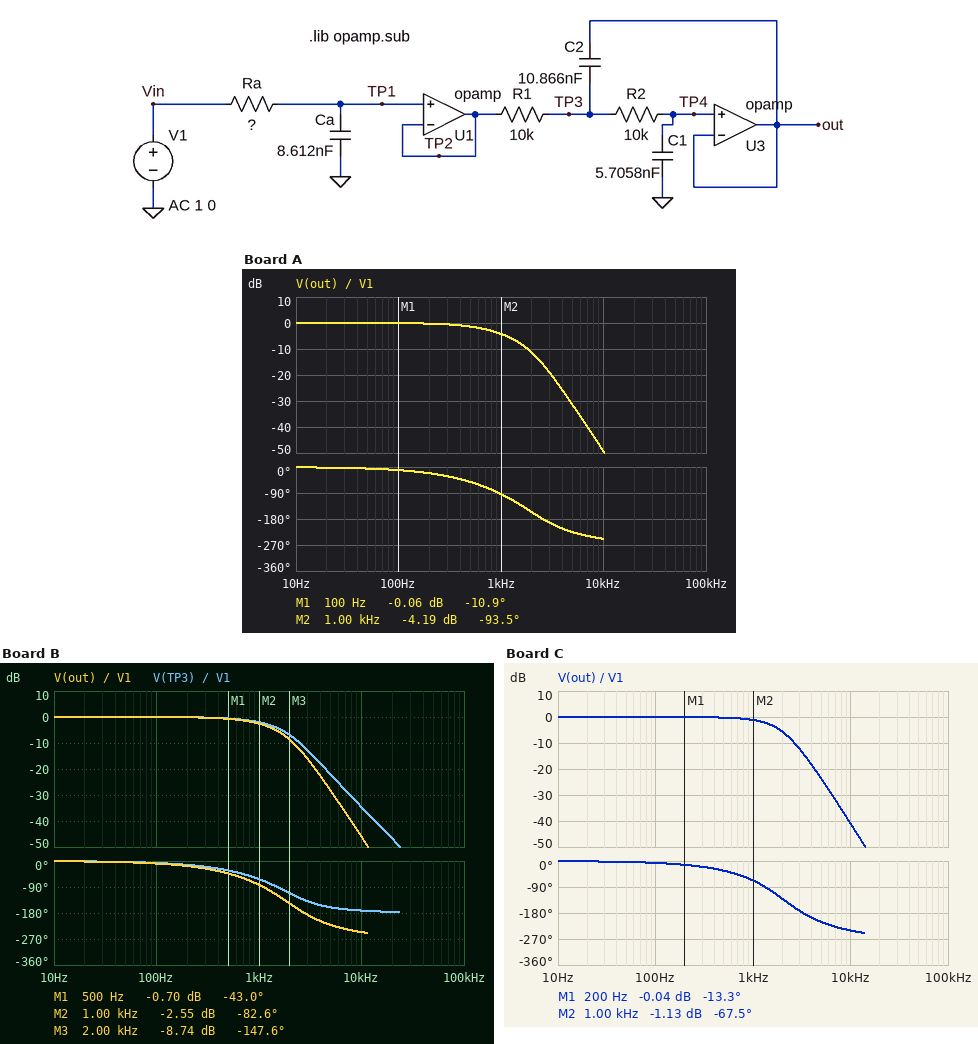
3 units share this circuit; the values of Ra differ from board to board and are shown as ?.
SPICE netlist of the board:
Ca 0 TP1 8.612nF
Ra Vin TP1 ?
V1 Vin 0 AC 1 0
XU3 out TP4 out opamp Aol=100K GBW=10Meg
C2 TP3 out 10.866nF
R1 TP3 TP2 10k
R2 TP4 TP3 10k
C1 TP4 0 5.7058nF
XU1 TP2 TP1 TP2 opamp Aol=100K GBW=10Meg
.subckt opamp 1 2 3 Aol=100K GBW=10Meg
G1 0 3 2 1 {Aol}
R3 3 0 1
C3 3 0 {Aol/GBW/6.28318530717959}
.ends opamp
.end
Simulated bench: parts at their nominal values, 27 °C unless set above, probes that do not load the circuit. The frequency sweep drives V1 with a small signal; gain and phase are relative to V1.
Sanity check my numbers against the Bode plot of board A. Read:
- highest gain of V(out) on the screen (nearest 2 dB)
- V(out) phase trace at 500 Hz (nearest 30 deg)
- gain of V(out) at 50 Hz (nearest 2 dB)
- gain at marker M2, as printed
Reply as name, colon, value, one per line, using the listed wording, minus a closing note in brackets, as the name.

highest gain of V(out) on the screen: 0 dB
V(out) phase trace at 500 Hz: -60 deg
gain of V(out) at 50 Hz: 0 dB
gain at marker M2, as printed: -4.19 dB
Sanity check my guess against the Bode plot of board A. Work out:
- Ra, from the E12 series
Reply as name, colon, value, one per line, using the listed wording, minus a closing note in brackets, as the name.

Ra, from the E12 series: 22 kΩ
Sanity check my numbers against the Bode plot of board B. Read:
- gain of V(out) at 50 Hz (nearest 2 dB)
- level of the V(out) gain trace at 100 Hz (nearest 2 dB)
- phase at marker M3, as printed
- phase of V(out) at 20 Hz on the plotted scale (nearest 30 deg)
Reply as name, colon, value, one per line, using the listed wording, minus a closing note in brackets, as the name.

gain of V(out) at 50 Hz: 0 dB
level of the V(out) gain trace at 100 Hz: 0 dB
phase at marker M3, as printed: -147.6 deg
phase of V(out) at 20 Hz on the plotted scale: 0 deg
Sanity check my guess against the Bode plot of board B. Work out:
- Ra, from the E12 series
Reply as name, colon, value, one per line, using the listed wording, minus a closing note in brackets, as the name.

Ra, from the E12 series: 15 kΩ
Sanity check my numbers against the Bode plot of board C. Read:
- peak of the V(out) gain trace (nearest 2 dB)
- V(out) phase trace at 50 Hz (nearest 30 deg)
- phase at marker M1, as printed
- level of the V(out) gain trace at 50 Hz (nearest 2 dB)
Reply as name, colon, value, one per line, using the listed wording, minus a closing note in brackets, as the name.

peak of the V(out) gain trace: 0 dB
V(out) phase trace at 50 Hz: 0 deg
phase at marker M1, as printed: -13.3 deg
level of the V(out) gain trace at 50 Hz: 0 dB
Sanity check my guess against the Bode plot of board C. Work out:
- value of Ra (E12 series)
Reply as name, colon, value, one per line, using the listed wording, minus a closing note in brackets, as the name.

value of Ra: 8.2 kΩ
